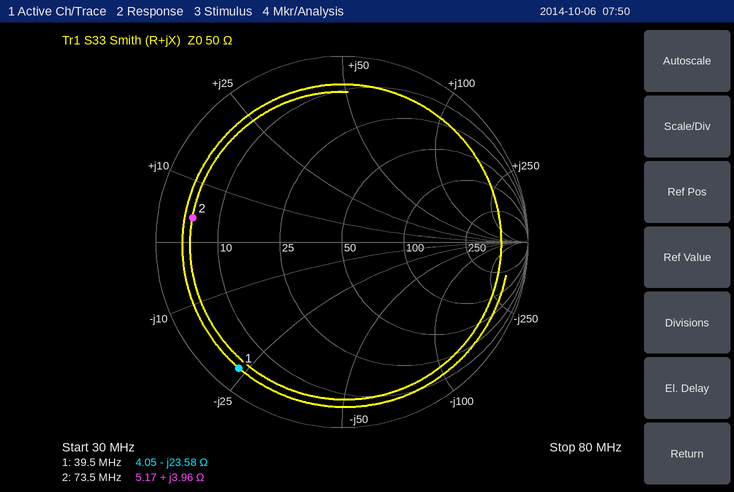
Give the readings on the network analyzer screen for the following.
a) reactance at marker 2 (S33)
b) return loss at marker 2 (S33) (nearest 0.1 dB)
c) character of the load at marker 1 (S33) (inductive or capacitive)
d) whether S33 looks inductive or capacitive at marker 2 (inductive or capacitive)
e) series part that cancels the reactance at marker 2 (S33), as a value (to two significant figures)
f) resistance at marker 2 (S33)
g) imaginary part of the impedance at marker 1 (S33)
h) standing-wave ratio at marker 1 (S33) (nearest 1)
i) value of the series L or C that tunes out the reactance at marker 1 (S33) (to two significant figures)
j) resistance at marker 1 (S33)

+3.96 Ω
1.8 dB
capacitive
inductive
550 pF
5.17 Ω
-23.58 Ω
15
95 nH
4.05 Ω
